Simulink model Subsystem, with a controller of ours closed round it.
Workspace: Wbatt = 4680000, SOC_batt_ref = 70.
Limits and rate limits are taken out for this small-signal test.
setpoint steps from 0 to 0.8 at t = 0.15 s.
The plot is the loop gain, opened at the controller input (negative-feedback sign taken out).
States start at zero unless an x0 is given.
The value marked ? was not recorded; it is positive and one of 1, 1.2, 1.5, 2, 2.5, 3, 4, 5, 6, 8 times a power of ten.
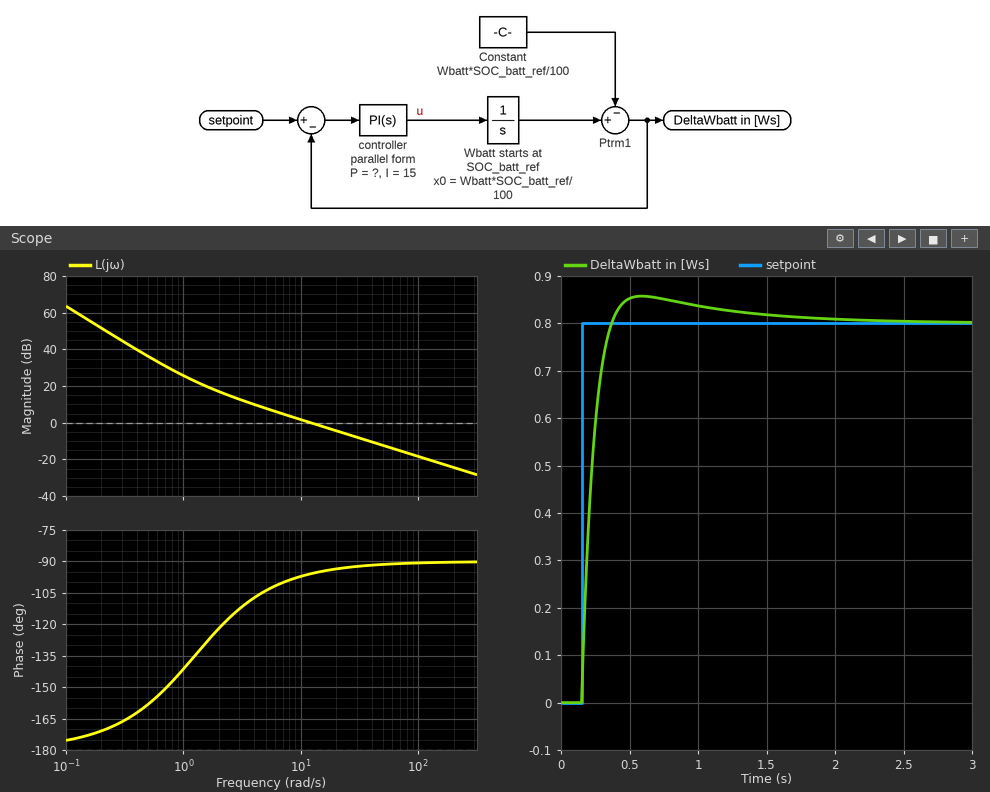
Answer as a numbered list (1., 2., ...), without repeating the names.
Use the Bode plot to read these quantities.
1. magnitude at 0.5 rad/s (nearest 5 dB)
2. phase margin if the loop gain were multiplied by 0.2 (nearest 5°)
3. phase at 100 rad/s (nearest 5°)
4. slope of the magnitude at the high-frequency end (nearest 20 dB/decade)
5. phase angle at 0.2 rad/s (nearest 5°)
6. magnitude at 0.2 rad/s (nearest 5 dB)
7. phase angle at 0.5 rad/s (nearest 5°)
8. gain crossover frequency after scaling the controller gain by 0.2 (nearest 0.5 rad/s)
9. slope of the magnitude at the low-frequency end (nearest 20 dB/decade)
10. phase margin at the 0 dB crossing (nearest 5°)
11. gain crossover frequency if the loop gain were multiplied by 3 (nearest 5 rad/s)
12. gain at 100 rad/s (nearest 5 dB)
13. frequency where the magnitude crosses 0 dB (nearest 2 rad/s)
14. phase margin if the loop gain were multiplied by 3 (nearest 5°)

1. 35 dB
2. 65°
3. -90°
4. -20 dB/decade
5. -170°
6. 50 dB
7. -160°
8. 2.5 rad/s
9. -40 dB/decade
10. 85°
11. 35 rad/s
12. -20 dB
13. 12 rad/s
14. 90°
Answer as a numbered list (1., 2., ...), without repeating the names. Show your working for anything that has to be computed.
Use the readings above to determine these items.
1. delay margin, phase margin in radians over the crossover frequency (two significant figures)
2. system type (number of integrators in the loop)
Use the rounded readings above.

1. 85 × π / 180 / 12 = 0.12 s
2. 2
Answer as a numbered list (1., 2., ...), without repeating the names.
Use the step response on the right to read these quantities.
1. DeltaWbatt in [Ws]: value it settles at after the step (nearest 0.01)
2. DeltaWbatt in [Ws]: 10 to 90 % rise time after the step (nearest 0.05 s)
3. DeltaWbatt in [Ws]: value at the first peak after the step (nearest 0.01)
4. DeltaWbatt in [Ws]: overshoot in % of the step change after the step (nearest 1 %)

1. 0.80
2. 0.15 s
3. 0.86
4. 7 %
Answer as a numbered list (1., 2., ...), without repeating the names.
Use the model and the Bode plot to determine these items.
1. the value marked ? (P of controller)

1. 12
